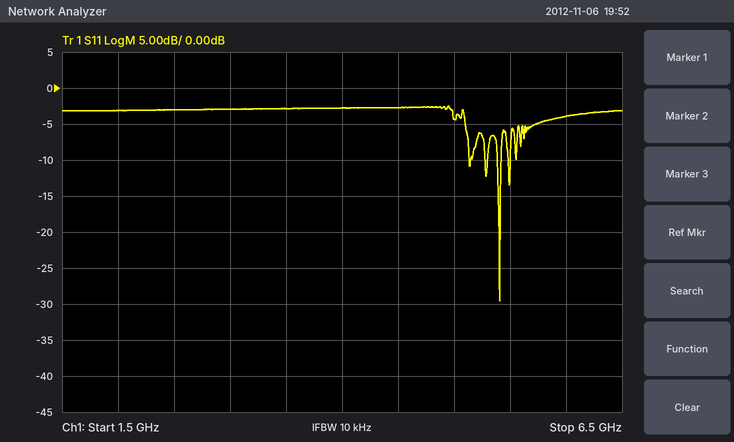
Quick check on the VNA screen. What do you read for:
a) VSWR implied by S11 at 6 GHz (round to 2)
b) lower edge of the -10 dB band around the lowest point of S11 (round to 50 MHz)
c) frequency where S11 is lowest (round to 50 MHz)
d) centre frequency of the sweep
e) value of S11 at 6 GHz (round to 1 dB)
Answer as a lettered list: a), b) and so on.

a) 4
b) 5.40 GHz
c) 5.40 GHz
d) 4 GHz
e) -4 dB
